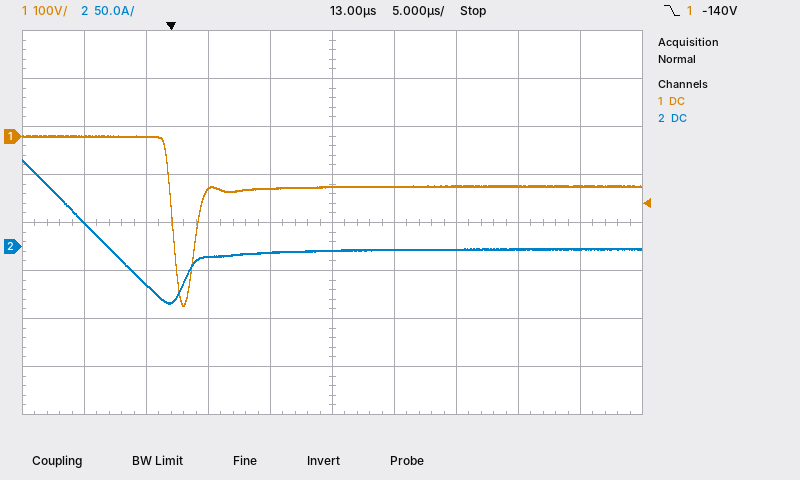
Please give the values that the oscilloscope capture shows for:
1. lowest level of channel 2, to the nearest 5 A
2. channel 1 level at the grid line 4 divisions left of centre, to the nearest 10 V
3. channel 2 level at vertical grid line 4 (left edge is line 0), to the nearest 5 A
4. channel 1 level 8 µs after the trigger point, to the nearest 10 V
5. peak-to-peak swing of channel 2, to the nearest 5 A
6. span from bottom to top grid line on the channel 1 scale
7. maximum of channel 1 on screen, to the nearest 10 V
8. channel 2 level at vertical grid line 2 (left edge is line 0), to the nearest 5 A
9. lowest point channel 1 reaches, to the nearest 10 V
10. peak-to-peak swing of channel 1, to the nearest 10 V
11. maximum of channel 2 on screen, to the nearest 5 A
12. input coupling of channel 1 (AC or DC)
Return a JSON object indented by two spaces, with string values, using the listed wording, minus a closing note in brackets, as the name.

{
  "lowest level of channel 2, to the nearest 5 A": "-60 A",
  "channel 1 level at the grid line 4 divisions left of centre, to the nearest 10 V": "0 V",
  "channel 2 level at vertical grid line 4 (left edge is line 0), to the nearest 5 A": "-5 A",
  "channel 1 level 8 µs after the trigger point, to the nearest 10 V": "-110 V",
  "peak-to-peak swing of channel 2, to the nearest 5 A": "150 A",
  "span from bottom to top grid line on the channel 1 scale": "800 V",
  "maximum of channel 1 on screen, to the nearest 10 V": "0 V",
  "channel 2 level at vertical grid line 2 (left edge is line 0), to the nearest 5 A": "-40 A",
  "lowest point channel 1 reaches, to the nearest 10 V": "-350 V",
  "peak-to-peak swing of channel 1, to the nearest 10 V": "350 V",
  "maximum of channel 2 on screen, to the nearest 5 A": "90 A",
  "input coupling of channel 1": "DC"
}
